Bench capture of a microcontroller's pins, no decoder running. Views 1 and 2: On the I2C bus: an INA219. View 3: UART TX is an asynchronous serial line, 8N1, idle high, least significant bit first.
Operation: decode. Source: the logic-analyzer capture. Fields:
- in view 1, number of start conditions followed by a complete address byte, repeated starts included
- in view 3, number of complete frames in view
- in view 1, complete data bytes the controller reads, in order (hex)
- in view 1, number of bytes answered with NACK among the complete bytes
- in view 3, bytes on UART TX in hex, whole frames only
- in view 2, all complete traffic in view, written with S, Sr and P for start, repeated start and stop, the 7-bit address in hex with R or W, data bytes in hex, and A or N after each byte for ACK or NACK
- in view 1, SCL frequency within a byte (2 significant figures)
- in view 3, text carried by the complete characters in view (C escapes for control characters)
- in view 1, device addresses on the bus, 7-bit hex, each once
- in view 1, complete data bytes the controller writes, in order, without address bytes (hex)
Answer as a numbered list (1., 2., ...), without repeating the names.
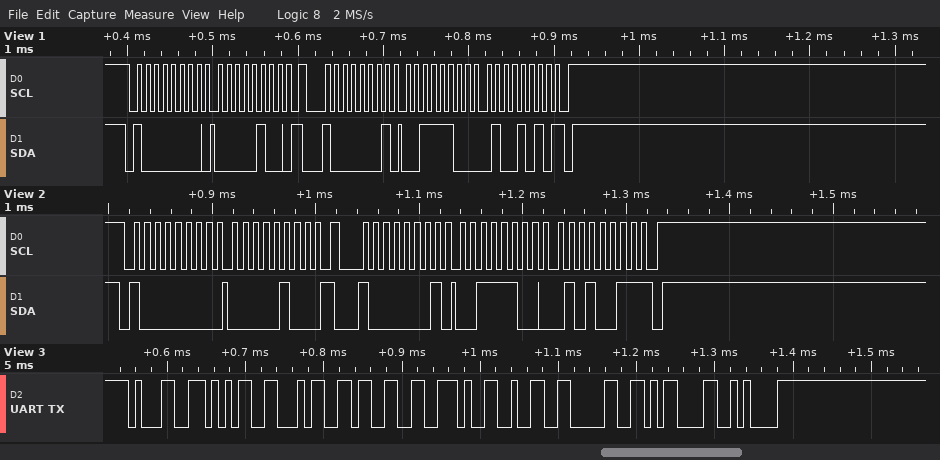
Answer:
1. 2
2. 9
3. 3C 4A
4. 1
5. 31 35 34 33 2E 32 30 0D 0A
6. S 40W A 04 A Sr 40R A 3C A 53 N P
7. 100 kHz
8. "1543.20\r\n"
9. 0x40
10. 04
